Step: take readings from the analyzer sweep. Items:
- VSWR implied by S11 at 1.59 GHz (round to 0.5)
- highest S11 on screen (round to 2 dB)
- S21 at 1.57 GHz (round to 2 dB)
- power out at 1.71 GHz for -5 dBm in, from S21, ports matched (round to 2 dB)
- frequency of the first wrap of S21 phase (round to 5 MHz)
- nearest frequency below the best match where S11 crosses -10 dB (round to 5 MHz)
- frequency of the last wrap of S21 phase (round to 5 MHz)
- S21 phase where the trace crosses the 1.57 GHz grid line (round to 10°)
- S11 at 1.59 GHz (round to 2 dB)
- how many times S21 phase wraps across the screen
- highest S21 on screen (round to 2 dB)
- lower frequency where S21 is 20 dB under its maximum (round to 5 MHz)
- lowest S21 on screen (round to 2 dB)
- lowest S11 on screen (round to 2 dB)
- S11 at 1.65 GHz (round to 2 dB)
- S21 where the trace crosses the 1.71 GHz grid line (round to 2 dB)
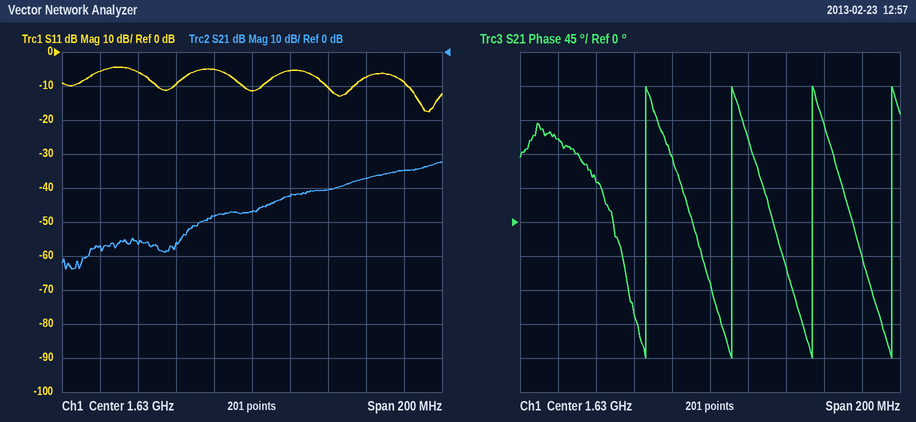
2.0
-4 dB
-56 dB
-40 dBm
1.595 GHz
1.710 GHz
1.725 GHz
50°
-10 dB
4
-32 dB
1.595 GHz
-64 dB
-18 dB
-6 dB
-34 dB
